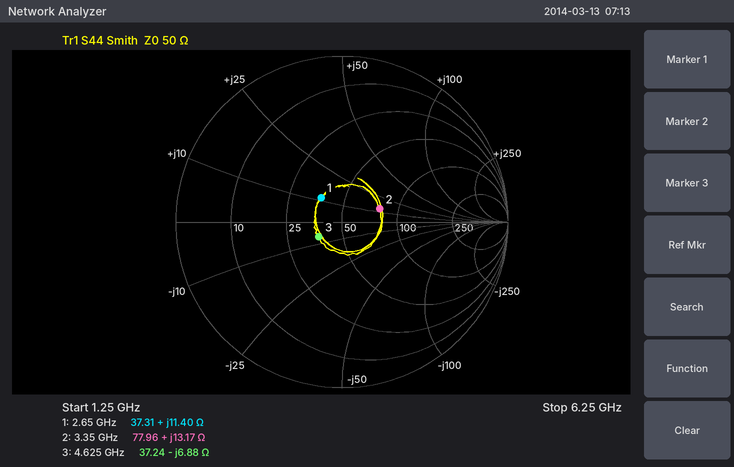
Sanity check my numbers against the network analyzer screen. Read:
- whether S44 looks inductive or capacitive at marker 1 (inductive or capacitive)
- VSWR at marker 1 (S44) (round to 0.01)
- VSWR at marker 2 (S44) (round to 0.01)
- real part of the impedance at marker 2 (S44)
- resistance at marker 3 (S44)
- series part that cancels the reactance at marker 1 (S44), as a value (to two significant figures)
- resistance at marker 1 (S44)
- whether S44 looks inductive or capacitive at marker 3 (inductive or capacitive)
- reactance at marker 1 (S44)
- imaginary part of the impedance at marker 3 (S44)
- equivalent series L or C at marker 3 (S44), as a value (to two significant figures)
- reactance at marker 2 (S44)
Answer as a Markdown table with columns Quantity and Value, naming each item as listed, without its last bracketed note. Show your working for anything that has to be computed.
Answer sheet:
| Quantity | Value |
|---|---|
| whether S44 looks inductive or capacitive at marker 1 | inductive |
| VSWR at marker 1 (S44) | 1.48 |
| VSWR at marker 2 (S44) | 1.63 |
| real part of the impedance at marker 2 | 77.96 Ω |
| resistance at marker 3 | 37.24 Ω |
| series part that cancels the reactance at marker 1 (S44), as a value | C = 1/(2π × 2.65 GHz × 11.4 Ω) ≈ 5.3 pF |
| resistance at marker 1 | 37.31 Ω |
| whether S44 looks inductive or capacitive at marker 3 | capacitive |
| reactance at marker 1 | +11.40 Ω |
| imaginary part of the impedance at marker 3 | -6.88 Ω |
| equivalent series L or C at marker 3 (S44), as a value | C = 1/(2π × 4.625 GHz × 6.88 Ω) ≈ 5.0 pF |
| reactance at marker 2 | +13.17 Ω |
